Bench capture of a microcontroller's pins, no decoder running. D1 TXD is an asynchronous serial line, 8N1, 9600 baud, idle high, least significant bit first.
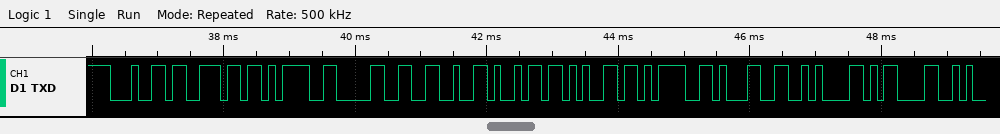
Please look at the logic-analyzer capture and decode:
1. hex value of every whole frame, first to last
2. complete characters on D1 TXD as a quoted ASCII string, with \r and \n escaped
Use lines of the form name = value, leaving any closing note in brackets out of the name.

hex value of every whole frame, first to last = 0x64 0x6E 0x3D 0x30 0x26 0x69 0x65 0x3D 0x31 0x0A 0x0D
complete characters on D1 TXD as a quoted ASCII string, with \r and \n escaped = "dn=0&ie=1\n\r"
